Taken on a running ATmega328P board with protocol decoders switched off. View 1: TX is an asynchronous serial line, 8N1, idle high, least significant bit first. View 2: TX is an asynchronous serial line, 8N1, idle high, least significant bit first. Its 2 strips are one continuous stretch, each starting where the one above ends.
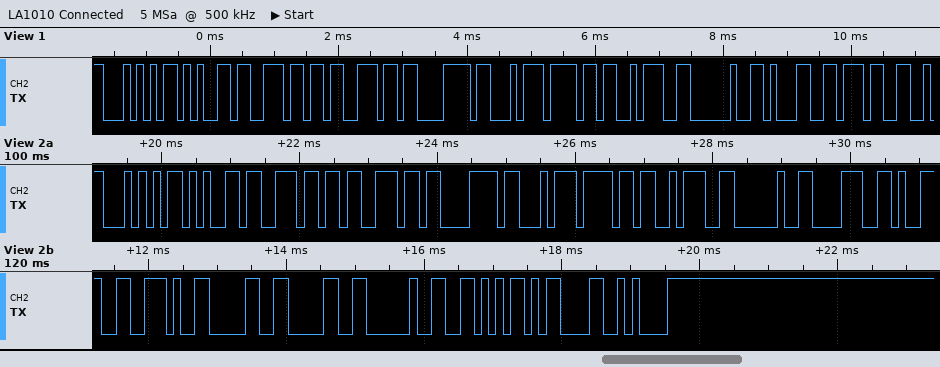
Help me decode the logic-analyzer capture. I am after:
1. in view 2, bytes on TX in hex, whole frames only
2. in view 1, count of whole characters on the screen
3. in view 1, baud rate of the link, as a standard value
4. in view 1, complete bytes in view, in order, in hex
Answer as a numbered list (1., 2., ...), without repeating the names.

1. 54 65 6E 73 C3 A3 6F 3A 20 38 39 2E 30 30 20 56 0D 0A
2. 11
3. 9600 baud
4. 54 65 6E 73 C3 A3 6F 3A 20 31 37
